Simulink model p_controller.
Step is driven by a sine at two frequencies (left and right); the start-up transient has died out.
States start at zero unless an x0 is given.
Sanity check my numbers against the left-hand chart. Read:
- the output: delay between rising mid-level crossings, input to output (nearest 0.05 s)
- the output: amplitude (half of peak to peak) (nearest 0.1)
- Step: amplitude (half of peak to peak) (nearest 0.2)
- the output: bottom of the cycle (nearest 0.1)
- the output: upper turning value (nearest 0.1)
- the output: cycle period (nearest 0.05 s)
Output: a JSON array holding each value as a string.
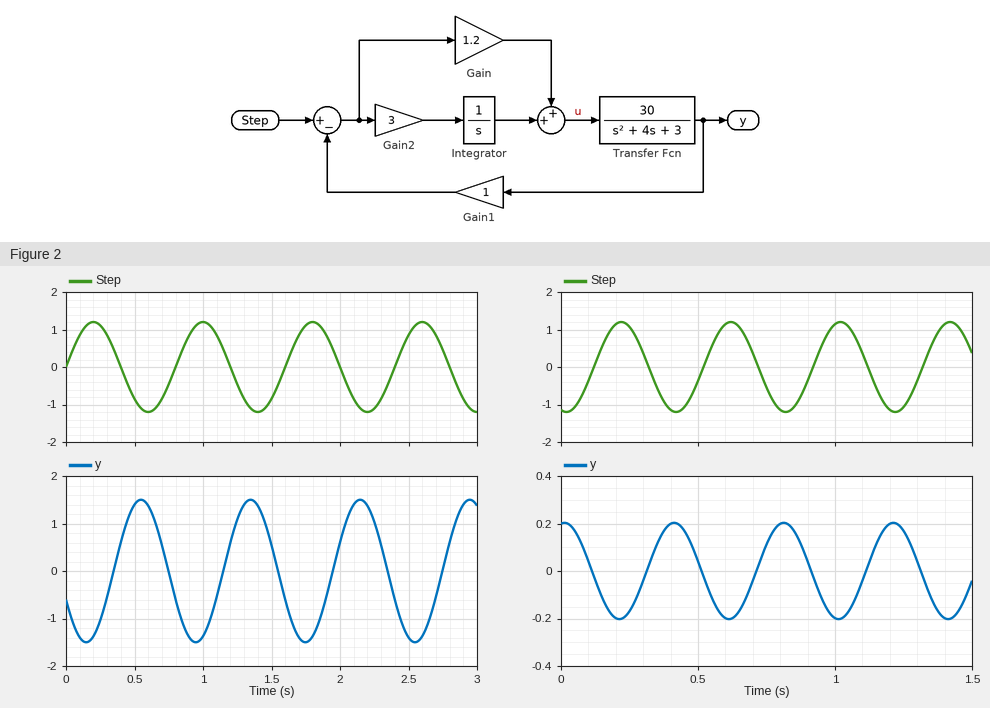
["0.35 s", "1.5", "1.2", "-1.5", "1.5", "0.80 s"]
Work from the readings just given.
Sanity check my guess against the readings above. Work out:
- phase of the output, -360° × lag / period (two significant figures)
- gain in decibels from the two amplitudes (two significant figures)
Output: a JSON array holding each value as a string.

["-160°", "1.9 dB"]
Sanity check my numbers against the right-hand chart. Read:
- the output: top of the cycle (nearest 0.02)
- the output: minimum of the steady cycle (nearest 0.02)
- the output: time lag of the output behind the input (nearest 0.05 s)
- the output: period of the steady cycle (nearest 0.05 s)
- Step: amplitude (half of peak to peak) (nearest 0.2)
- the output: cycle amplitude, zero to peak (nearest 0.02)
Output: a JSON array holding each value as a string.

["0.20", "-0.20", "0.20 s", "0.40 s", "1.2", "0.20"]
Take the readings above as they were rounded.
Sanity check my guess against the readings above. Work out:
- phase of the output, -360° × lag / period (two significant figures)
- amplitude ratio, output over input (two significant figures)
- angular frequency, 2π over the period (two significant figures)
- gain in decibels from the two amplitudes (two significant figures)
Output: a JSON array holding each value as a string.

["-180°", "0.17", "16 rad/s", "-16 dB"]
